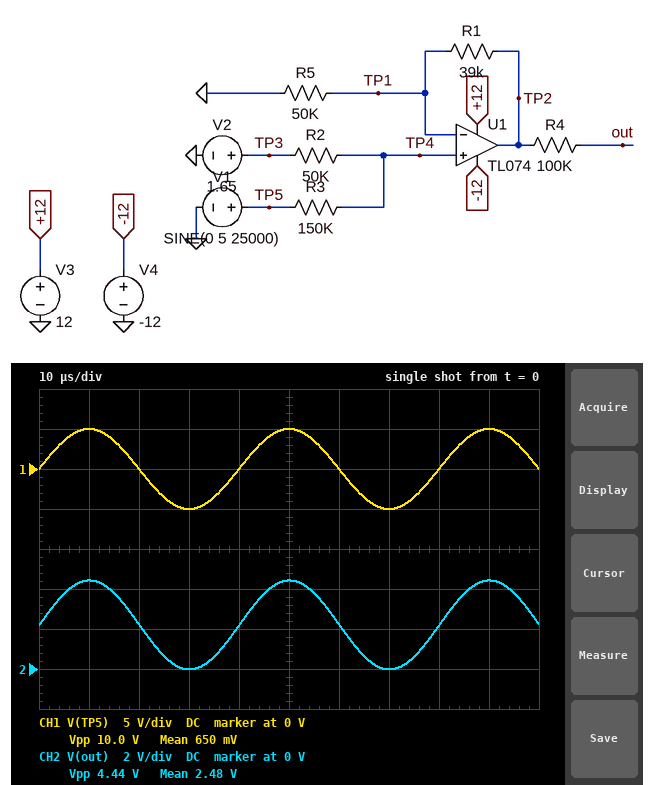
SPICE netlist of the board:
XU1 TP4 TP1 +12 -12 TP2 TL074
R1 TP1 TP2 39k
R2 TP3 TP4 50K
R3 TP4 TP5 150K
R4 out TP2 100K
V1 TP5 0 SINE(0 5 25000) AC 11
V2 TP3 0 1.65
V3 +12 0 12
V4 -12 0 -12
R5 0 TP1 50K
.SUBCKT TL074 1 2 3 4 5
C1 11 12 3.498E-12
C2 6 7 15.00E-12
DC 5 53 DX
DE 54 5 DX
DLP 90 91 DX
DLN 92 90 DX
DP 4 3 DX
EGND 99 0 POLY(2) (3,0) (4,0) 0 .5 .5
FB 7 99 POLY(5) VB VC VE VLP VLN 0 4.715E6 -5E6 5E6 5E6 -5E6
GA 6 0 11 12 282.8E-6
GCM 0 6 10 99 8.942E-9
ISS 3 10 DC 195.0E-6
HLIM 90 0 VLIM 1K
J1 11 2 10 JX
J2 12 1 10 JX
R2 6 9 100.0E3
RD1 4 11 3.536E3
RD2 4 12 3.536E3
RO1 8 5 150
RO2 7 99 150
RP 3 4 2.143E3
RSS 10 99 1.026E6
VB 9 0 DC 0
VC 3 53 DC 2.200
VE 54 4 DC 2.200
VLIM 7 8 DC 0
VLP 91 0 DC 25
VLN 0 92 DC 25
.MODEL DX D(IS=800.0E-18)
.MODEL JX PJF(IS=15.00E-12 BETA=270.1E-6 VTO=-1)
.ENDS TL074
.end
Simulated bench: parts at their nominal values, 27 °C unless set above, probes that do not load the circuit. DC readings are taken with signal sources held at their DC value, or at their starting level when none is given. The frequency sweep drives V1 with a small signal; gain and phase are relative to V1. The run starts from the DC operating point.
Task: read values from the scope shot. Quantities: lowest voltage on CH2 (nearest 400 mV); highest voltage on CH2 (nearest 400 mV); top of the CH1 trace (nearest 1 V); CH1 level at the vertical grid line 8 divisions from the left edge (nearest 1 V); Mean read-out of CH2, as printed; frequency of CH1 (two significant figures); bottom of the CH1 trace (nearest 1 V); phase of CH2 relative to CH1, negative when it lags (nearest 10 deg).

0 V
4.4 V
5 V
0 V
2.48 V
25 kHz
-5 V
0 deg
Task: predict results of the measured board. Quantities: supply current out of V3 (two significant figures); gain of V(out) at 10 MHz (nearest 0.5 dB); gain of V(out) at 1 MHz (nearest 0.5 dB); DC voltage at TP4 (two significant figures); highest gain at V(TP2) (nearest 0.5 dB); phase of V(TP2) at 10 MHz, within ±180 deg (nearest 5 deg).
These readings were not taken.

11 mA
-26.0 dB
-7.5 dB
1.2 V
-7.0 dB
-145 deg
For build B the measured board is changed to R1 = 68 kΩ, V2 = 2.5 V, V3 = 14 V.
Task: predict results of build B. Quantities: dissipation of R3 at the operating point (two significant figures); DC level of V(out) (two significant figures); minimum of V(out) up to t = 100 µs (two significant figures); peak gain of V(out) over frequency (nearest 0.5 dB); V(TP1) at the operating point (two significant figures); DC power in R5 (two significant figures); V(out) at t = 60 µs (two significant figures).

23 µW
4.4 V
1.5 V
-4.5 dB
1.9 V
70 µW
4.5 V
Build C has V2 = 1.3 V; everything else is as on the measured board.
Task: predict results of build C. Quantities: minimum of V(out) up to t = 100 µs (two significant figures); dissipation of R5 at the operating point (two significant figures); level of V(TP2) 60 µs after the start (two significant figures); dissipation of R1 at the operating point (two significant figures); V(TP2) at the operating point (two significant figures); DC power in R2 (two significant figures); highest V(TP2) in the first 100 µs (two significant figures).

-490 mV
19 µW
1.8 V
15 µW
1.7 V
2.1 µW
4.0 V
